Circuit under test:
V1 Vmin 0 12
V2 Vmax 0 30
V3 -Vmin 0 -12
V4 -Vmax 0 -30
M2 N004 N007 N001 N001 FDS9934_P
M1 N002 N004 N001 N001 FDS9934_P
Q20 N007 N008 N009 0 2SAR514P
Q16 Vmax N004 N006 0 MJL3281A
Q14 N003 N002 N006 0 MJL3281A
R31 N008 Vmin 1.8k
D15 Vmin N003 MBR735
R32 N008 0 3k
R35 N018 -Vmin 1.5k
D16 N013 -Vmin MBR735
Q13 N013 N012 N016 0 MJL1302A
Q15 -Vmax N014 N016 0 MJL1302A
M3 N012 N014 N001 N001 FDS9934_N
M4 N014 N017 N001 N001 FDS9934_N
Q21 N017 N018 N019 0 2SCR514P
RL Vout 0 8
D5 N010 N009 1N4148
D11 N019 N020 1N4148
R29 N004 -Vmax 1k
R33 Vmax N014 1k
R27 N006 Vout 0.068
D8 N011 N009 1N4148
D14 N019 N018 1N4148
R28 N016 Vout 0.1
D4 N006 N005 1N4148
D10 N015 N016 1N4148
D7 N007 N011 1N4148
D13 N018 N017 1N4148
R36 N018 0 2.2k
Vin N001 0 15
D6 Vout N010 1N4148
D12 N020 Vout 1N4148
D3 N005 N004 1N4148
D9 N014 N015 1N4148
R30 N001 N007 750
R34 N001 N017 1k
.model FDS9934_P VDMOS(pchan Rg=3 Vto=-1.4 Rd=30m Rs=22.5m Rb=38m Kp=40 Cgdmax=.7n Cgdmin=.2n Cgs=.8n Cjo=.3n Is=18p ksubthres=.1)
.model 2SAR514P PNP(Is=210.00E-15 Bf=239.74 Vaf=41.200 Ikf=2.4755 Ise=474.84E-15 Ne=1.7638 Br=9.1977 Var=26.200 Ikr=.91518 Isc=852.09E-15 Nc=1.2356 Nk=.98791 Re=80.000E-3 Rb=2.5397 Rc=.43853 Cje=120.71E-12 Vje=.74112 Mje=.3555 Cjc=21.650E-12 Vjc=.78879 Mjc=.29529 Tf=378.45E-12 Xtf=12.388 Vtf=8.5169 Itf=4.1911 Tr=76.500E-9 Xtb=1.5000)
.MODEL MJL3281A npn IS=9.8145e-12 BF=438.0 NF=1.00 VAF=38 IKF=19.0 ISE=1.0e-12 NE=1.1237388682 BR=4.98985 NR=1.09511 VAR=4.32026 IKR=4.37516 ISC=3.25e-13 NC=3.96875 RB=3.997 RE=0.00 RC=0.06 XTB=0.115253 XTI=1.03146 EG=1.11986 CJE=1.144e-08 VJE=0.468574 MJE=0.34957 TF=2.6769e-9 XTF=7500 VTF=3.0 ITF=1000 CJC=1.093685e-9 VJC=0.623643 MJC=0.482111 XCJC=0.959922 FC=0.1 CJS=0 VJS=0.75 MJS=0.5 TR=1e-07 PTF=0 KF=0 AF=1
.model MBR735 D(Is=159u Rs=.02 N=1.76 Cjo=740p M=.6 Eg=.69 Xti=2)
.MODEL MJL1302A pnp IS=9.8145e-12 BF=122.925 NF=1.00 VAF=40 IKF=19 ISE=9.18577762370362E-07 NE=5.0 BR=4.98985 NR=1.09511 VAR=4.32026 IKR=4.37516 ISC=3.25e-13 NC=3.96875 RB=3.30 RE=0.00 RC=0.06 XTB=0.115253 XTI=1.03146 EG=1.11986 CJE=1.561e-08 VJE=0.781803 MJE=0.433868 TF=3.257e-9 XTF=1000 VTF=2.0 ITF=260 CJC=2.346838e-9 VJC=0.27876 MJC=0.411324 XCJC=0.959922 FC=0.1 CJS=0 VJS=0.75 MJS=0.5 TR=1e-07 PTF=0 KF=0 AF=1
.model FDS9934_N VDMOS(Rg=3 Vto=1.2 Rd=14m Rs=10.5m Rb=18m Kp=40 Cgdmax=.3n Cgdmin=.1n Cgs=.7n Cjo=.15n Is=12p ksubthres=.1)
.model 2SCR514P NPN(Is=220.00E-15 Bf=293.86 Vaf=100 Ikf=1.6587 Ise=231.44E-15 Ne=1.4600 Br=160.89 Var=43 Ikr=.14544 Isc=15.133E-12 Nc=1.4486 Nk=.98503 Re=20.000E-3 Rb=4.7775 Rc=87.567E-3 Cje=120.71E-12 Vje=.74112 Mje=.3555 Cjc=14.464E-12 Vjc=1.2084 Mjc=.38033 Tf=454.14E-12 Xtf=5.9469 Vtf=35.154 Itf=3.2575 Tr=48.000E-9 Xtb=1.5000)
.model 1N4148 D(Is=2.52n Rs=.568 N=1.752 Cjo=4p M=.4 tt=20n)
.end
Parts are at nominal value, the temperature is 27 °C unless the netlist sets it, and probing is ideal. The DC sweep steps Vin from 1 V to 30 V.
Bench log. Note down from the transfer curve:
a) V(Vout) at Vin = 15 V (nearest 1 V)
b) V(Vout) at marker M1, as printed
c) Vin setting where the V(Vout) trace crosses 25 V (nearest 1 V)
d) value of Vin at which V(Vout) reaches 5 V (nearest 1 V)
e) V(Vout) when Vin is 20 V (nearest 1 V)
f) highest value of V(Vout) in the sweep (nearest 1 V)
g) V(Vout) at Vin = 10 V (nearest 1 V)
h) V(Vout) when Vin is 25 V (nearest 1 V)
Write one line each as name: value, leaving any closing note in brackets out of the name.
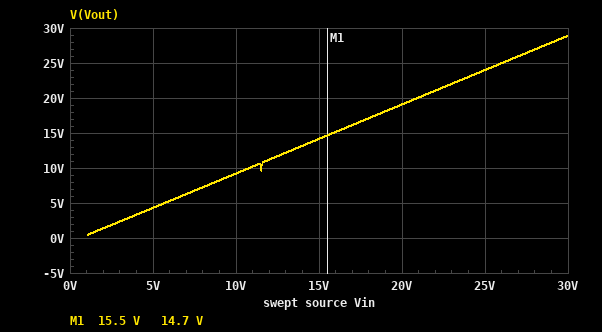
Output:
V(Vout) at Vin = 15 V: 14 V
V(Vout) at marker M1, as printed: 14.7 V
Vin setting where the V(Vout) trace crosses 25 V: 26 V
value of Vin at which V(Vout) reaches 5 V: 6 V
V(Vout) when Vin is 20 V: 19 V
highest value of V(Vout) in the sweep: 29 V
V(Vout) at Vin = 10 V: 9 V
V(Vout) when Vin is 25 V: 24 V
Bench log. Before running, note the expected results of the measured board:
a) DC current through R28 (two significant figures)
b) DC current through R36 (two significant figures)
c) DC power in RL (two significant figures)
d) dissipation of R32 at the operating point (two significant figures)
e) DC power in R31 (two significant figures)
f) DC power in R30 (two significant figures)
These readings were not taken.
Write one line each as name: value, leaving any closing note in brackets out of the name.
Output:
DC current through R28: 14 mA
DC current through R36: 3.2 mA
DC power in RL: 25 W
dissipation of R32 at the operating point: 50 mW
DC power in R31: 42 µW
DC power in R30: 5.6 mW
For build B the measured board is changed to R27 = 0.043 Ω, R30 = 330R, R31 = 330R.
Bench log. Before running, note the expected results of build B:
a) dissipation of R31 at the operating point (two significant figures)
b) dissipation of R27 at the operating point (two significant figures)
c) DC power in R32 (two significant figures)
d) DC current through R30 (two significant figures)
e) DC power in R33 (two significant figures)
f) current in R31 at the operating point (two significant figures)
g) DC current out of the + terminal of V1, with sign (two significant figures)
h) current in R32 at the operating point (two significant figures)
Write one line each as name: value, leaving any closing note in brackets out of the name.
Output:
dissipation of R31 at the operating point: 750 µW
dissipation of R27 at the operating point: 130 mW
DC power in R32: 52 mW
DC current through R30: 5.5 mA
DC power in R33: 210 mW
current in R31 at the operating point: 1.5 mA
DC current out of the + terminal of V1, with sign: -1.5 mA
current in R32 at the operating point: 4.2 mA
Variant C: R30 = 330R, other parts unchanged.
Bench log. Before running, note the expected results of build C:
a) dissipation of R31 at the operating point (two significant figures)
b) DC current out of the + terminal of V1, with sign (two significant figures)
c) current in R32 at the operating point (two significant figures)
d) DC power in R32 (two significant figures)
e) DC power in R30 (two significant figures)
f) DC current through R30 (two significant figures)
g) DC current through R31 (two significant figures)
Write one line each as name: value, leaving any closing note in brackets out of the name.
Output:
dissipation of R31 at the operating point: 330 µW
DC current out of the + terminal of V1, with sign: -430 µA
current in R32 at the operating point: 4.3 mA
DC power in R32: 54 mW
DC power in R30: 7.2 mW
DC current through R30: 4.7 mA
DC current through R31: 430 µA
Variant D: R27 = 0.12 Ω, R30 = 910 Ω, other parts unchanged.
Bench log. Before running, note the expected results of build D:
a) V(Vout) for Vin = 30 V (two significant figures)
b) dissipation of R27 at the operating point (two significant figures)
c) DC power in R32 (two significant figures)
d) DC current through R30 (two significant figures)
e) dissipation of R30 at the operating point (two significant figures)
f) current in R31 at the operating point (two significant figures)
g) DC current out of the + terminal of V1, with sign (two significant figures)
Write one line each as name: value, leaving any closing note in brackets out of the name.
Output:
V(Vout) for Vin = 30 V: 29 V
dissipation of R27 at the operating point: 370 mW
DC power in R32: 49 mW
DC current through R30: 2.4 mA
dissipation of R30 at the operating point: 5.1 mW
current in R31 at the operating point: 95 µA
DC current out of the + terminal of V1, with sign: -95 µA
